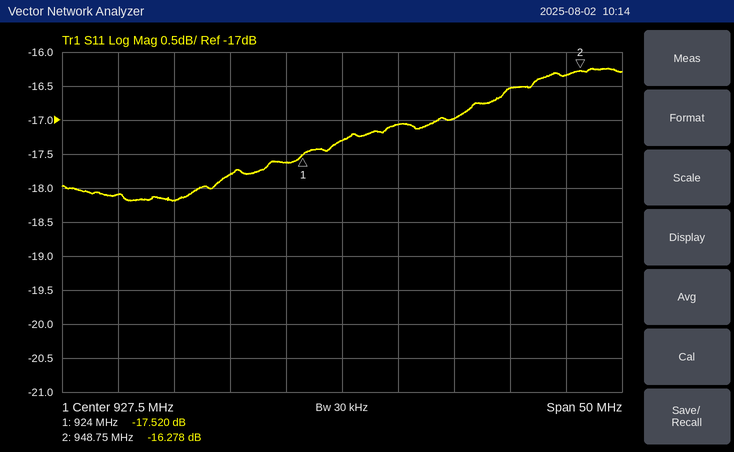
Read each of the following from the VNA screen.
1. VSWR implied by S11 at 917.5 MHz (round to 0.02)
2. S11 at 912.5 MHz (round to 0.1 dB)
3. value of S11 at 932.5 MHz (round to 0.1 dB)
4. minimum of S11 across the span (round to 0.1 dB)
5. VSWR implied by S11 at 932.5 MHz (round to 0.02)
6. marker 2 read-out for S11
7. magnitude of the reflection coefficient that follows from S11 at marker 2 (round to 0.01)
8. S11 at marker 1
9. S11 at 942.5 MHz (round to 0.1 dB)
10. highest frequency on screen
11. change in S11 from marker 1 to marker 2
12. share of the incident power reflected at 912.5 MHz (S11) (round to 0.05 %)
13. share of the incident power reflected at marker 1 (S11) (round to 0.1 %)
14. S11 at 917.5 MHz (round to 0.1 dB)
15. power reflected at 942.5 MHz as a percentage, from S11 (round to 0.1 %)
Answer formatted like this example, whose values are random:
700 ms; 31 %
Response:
1.30; -18.2 dB; -17.1 dB; -18.2 dB; 1.32; -16.278 dB; 0.15; -17.520 dB; -16.5 dB; 952.5 MHz; 1.242 dB; 1.50 %; 1.8 %; -17.8 dB; 2.2 %
